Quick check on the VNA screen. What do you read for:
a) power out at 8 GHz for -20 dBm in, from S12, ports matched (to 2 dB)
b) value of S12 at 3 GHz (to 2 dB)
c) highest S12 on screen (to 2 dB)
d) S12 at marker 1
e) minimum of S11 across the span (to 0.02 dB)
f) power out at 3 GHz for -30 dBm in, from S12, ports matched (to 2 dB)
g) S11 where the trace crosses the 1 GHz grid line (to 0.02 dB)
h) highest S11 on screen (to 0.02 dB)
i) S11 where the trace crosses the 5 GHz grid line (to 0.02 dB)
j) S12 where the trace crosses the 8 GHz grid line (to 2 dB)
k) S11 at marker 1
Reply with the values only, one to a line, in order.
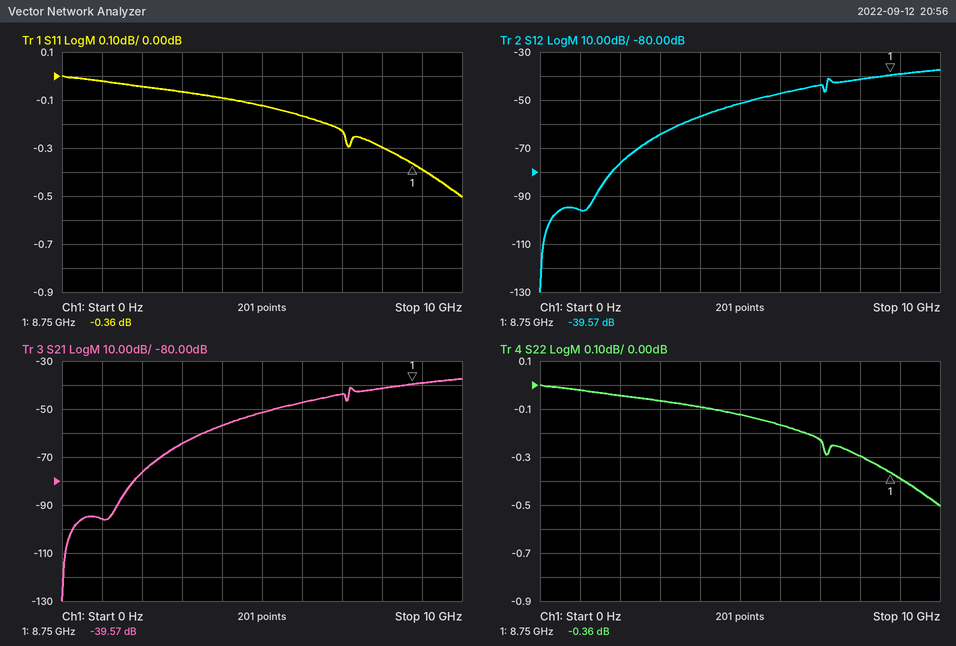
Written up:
-62 dBm
-64 dB
-38 dB
-39.57 dB
-0.50 dB
-94 dBm
-0.02 dB
0.00 dB
-0.12 dB
-42 dB
-0.36 dB
